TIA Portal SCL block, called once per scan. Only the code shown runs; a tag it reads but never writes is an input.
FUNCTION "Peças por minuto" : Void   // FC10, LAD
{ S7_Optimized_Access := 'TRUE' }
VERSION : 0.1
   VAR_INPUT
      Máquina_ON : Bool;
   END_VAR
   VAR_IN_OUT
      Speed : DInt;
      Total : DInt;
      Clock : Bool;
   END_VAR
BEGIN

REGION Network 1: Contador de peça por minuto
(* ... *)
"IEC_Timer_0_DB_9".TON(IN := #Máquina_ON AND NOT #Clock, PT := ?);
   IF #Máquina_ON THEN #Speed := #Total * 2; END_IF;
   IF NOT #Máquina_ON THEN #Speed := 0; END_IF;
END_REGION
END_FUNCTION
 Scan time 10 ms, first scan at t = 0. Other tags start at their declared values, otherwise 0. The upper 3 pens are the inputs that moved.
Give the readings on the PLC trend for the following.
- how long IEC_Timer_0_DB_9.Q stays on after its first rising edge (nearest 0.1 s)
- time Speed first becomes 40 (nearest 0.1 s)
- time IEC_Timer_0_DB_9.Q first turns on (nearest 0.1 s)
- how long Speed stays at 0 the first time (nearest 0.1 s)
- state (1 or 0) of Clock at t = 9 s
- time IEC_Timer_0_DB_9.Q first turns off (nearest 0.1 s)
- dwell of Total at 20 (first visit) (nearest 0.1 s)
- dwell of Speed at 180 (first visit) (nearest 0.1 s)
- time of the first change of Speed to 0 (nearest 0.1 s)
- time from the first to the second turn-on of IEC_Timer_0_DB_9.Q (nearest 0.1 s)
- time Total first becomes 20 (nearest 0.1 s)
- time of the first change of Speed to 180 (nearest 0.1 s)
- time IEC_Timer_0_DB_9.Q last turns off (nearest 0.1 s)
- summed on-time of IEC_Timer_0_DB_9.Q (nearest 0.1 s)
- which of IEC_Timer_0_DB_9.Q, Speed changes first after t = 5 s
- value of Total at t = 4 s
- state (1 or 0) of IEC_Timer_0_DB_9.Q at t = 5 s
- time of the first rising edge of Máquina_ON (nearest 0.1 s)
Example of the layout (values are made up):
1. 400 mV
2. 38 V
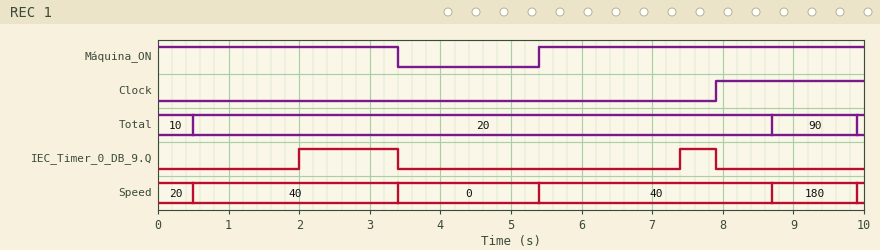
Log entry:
1. 1.4 s
2. 0.5 s
3. 2.0 s
4. 2.0 s
5. 1
6. 3.4 s
7. 8.2 s
8. 1.2 s
9. 3.4 s
10. 5.4 s
11. 0.5 s
12. 8.7 s
13. 7.9 s
14. 1.9 s
15. Speed
16. 20
17. 0
18. 5.4 s
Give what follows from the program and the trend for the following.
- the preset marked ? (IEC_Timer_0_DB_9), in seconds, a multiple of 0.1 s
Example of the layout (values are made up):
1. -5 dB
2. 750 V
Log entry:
1. 2.0 s
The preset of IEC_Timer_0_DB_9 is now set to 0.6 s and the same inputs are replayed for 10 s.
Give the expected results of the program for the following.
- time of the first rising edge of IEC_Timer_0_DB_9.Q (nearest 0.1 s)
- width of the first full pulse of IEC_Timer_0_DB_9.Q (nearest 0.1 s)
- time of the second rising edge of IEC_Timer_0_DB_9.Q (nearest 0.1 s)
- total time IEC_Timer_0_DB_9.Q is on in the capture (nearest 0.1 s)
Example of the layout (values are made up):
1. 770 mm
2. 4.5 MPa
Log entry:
1. 0.6 s
2. 2.8 s
3. 6.0 s
4. 4.7 s
